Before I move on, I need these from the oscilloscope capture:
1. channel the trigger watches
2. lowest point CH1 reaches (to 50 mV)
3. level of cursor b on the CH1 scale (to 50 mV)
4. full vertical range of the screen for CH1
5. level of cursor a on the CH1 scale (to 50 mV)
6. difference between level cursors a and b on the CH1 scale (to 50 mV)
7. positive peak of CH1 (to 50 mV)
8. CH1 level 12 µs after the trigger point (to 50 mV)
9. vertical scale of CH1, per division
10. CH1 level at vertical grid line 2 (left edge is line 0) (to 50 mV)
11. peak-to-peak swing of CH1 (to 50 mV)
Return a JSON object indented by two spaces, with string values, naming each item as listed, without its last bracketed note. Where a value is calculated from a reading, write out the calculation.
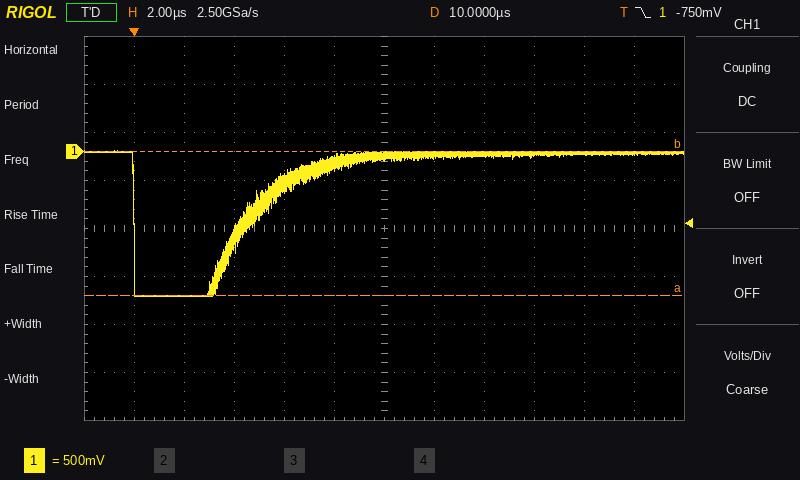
{
  "channel the trigger watches": "CH1",
  "lowest point CH1 reaches": "-1.50 V",
  "level of cursor b on the CH1 scale": "0 mV",
  "full vertical range of the screen for CH1": "4 V",
  "level of cursor a on the CH1 scale": "-1.50 V",
  "difference between level cursors a and b on the CH1 scale": "1.50 V",
  "positive peak of CH1": "0 mV",
  "CH1 level 12 µs after the trigger point": "-50 mV",
  "vertical scale of CH1, per division": "500 mV",
  "CH1 level at vertical grid line 2 (left edge is line 0)": "-1.50 V",
  "peak-to-peak swing of CH1": "0 mV − (-1.50 V) = 1.50 V"
}
